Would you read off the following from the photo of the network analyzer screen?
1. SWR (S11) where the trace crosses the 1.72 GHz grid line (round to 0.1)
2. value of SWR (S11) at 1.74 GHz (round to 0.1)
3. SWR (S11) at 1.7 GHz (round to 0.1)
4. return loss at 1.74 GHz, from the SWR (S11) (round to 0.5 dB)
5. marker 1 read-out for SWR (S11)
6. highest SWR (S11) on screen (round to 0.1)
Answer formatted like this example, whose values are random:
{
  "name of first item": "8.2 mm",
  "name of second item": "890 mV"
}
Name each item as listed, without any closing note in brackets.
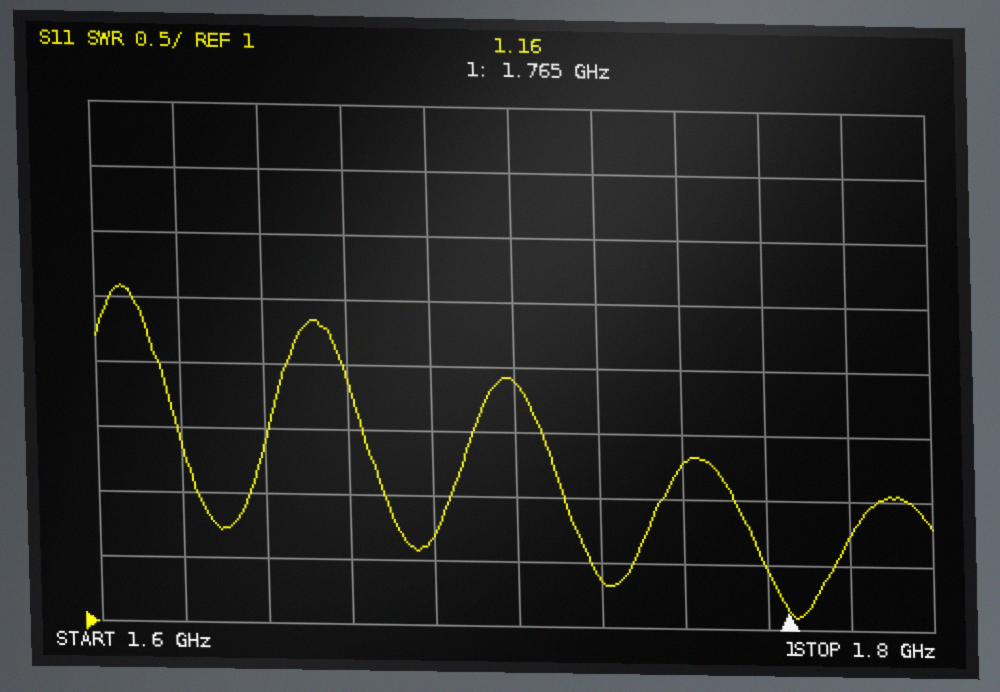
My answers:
{
  "SWR (S11) where the trace crosses the 1.72 GHz grid line": "1.4",
  "value of SWR (S11) at 1.74 GHz": "2.3",
  "SWR (S11) at 1.7 GHz": "2.9",
  "return loss at 1.74 GHz, from the SWR (S11)": "8.0 dB",
  "marker 1 read-out for SWR": "1.16",
  "highest SWR (S11) on screen": "3.6"
}
